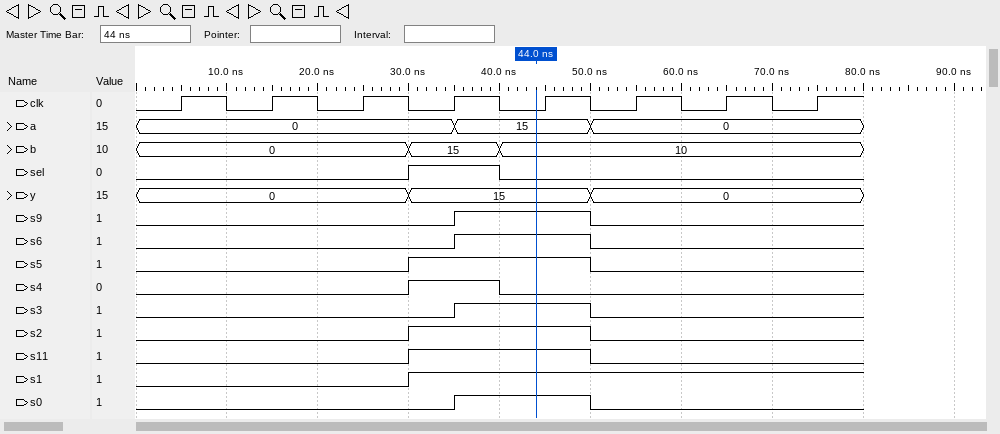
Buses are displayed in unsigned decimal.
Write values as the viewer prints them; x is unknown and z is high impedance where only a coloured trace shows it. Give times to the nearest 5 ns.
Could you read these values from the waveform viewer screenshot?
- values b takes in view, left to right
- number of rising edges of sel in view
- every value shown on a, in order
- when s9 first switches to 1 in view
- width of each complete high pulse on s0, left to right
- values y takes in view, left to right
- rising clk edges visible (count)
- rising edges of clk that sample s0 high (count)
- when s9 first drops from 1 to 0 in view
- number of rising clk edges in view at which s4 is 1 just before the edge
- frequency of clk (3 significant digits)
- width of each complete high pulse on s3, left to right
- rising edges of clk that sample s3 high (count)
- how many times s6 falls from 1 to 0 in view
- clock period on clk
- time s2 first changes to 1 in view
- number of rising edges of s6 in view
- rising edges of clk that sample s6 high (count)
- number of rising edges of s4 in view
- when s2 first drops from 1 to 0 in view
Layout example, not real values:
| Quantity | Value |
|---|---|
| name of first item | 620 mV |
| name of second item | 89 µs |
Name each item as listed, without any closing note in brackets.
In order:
| Quantity | Value |
|---|---|
| values b takes in view, left to right | 0, 15, 10 |
| number of rising edges of sel in view | 1 |
| every value shown on a, in order | 0, 15, 0 |
| when s9 first switches to 1 in view | 35 ns |
| width of each complete high pulse on s0, left to right | 15 ns |
| values y takes in view, left to right | 0, 15, 0 |
| rising clk edges visible | 8 |
| rising edges of clk that sample s0 high | 1 |
| when s9 first drops from 1 to 0 in view | 50 ns |
| number of rising clk edges in view at which s4 is 1 just before the edge | 1 |
| frequency of clk | 100 MHz |
| width of each complete high pulse on s3, left to right | 15 ns |
| rising edges of clk that sample s3 high | 1 |
| how many times s6 falls from 1 to 0 in view | 1 |
| clock period on clk | 10 ns |
| time s2 first changes to 1 in view | 30 ns |
| number of rising edges of s6 in view | 1 |
| rising edges of clk that sample s6 high | 1 |
| number of rising edges of s4 in view | 1 |
| when s2 first drops from 1 to 0 in view | 50 ns |
